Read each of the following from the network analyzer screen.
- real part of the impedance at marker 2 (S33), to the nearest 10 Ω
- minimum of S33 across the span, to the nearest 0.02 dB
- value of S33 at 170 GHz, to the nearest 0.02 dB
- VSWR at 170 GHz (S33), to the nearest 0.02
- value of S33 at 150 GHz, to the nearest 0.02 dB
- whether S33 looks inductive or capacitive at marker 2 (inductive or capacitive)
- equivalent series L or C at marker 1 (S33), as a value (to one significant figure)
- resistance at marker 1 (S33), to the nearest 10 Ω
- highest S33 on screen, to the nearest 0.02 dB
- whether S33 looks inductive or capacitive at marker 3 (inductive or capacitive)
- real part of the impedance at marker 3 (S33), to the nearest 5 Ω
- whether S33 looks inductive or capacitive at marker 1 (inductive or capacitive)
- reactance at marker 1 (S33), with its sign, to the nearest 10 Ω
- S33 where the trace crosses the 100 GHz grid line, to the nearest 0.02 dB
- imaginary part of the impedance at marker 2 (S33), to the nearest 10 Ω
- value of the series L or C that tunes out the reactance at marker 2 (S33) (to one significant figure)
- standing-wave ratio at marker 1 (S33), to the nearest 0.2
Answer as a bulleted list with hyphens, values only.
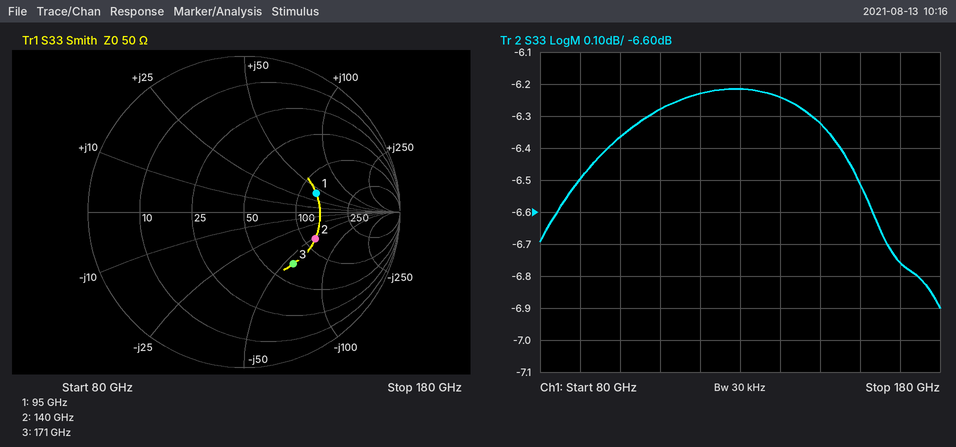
- 120 Ω
- -6.90 dB
- -6.76 dB
- 2.70
- -6.32 dB
- capacitive
- 70 pH
- 130 Ω
- -6.22 dB
- capacitive
- 70 Ω
- inductive
- +40 Ω
- -6.36 dB
- -50 Ω
- 60 pH
- 2.8
